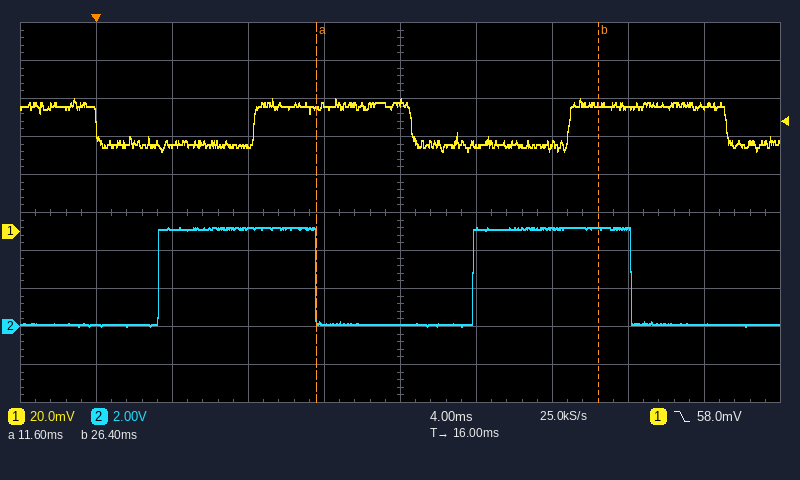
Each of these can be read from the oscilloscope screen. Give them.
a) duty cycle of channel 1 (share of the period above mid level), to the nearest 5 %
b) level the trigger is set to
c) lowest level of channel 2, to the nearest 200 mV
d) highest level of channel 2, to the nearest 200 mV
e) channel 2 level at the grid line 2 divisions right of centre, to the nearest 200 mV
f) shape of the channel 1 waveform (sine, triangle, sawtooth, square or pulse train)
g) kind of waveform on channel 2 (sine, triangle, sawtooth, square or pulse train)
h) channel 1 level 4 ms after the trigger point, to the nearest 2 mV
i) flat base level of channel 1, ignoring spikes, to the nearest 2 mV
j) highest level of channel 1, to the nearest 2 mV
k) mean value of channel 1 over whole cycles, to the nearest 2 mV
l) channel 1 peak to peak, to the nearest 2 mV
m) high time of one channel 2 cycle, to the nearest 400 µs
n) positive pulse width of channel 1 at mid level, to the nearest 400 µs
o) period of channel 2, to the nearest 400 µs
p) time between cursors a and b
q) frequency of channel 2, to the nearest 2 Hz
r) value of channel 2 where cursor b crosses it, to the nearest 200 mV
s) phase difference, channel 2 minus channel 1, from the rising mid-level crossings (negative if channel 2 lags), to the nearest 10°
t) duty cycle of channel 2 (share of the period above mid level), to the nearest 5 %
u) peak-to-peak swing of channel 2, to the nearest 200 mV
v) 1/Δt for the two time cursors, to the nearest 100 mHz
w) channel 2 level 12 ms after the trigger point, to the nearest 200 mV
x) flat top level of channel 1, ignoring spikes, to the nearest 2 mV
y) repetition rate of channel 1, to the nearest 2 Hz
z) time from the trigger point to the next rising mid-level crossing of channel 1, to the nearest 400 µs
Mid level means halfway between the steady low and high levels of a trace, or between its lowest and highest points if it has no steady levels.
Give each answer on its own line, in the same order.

50 %
58.0 mV
0.0 V
5.2 V
5.2 V
square
square
46 mV
46 mV
70 mV
56 mV
28 mV
8.4 ms
8.4 ms
16.4 ms
14.8 ms
60 Hz
5.2 V
+110°
50 %
5.2 V
67.6 Hz
200 mV
66 mV
60 Hz
8.4 ms
